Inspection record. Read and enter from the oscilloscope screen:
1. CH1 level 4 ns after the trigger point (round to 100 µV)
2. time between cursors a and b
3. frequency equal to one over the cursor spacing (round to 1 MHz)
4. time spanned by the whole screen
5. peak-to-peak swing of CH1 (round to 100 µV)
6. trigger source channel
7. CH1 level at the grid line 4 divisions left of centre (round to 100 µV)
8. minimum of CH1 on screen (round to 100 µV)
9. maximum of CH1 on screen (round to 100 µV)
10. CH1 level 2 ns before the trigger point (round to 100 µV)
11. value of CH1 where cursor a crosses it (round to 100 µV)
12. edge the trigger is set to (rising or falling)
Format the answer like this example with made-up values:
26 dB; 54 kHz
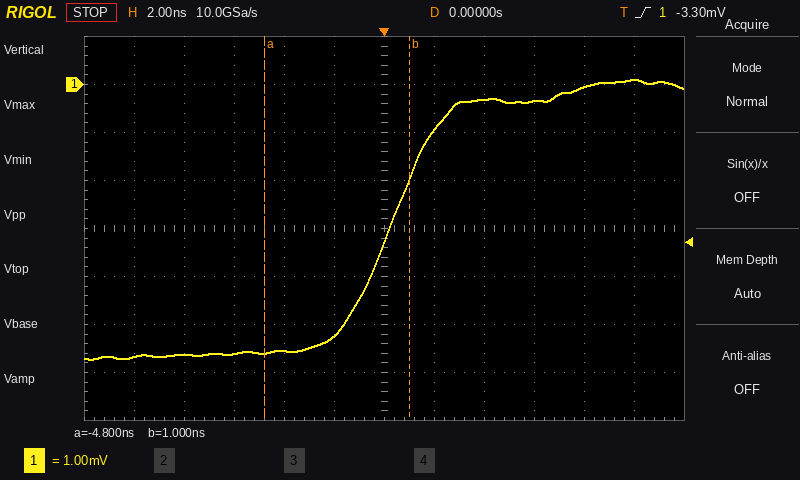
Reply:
-300 µV; 5.8 ns; 172 MHz; 24 ns; 5.8 mV; CH1; -5.6 mV; -5.7 mV; 100 µV; -5.2 mV; -5.6 mV; rising
